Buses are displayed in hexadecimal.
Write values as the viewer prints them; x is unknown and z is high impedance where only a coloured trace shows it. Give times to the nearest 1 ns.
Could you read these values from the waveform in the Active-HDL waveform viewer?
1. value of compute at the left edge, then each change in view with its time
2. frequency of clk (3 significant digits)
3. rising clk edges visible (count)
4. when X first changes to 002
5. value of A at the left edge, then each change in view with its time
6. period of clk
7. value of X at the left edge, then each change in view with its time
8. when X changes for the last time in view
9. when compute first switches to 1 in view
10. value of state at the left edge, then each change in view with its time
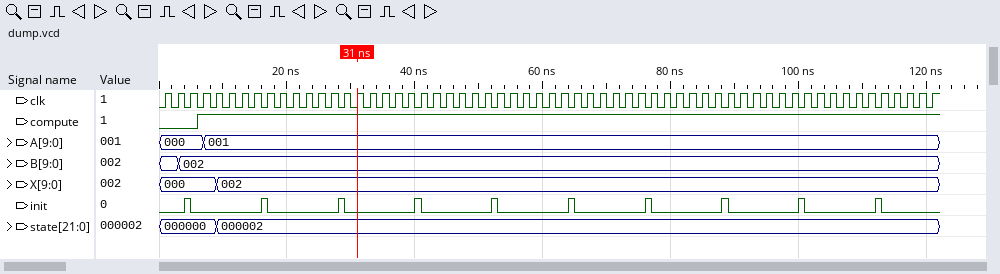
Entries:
0, 1 at 6 ns
500 MHz
61
9 ns
000, 001 at 7 ns
2 ns
000, 002 at 9 ns
9 ns
6 ns
000000, 000002 at 9 ns
